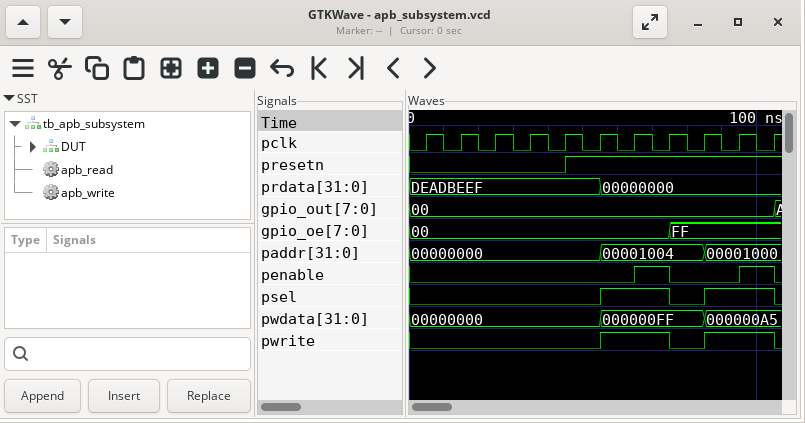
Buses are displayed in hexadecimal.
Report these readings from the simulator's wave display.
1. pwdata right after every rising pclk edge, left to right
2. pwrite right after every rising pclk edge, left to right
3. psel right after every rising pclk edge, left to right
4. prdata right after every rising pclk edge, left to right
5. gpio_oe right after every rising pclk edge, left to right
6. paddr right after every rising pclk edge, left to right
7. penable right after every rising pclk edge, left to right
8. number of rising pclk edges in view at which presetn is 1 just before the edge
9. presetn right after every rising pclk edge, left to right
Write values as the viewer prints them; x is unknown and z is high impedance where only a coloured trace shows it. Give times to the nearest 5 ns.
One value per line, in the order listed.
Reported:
00000000, 00000000, 00000000, 00000000, 00000000, 000000FF, 000000FF, 000000FF, 000000A5, 000000A5, 000000A5
0 0 0 0 0 1 1 0 1 1 0
0 0 0 0 0 1 1 0 1 1 0
DEADBEEF, DEADBEEF, DEADBEEF, DEADBEEF, DEADBEEF, 00000000, 00000000, 00000000, 00000000, 00000000, 00000000
00, 00, 00, 00, 00, 00, 00, FF, FF, FF, FF
00000000, 00000000, 00000000, 00000000, 00000000, 00001004, 00001004, 00001004, 00001000, 00001000, 00001000
0 0 0 0 0 0 1 0 0 1 0
6
0 0 0 0 1 1 1 1 1 1 1
